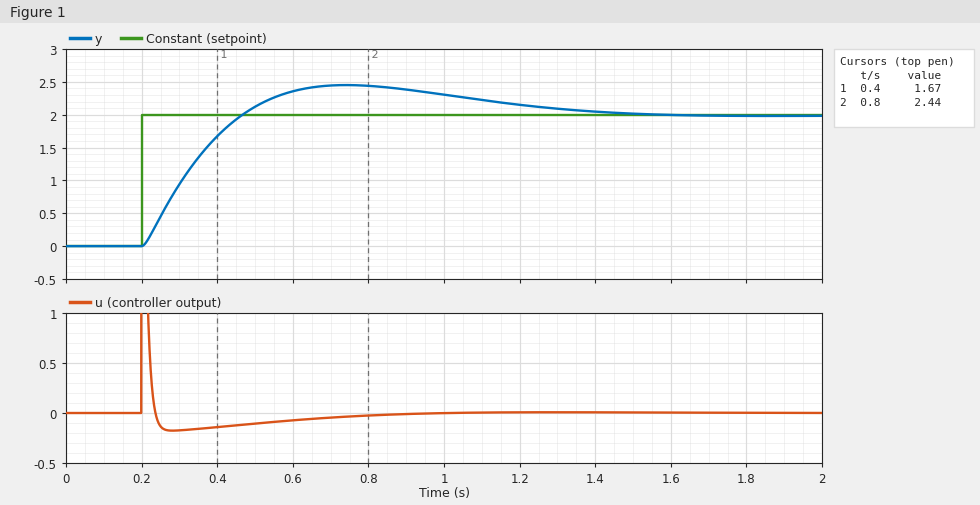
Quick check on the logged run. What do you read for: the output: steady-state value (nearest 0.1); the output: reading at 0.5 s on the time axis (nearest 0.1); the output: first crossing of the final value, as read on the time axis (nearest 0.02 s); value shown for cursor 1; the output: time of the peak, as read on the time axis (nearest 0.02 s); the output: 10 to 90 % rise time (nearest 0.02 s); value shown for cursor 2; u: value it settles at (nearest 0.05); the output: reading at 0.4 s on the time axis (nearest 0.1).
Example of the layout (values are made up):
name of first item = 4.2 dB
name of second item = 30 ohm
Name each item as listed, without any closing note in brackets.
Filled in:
the output: steady-state value = 2.0
the output: reading at 0.5 s on the time axis = 2.1
the output: first crossing of the final value, as read on the time axis = 0.46 s
value shown for cursor 1 = 1.67
the output: time of the peak, as read on the time axis = 0.74 s
the output: 10 to 90 % rise time = 0.20 s
value shown for cursor 2 = 2.44
u: value it settles at = 0.00
the output: reading at 0.4 s on the time axis = 1.7
